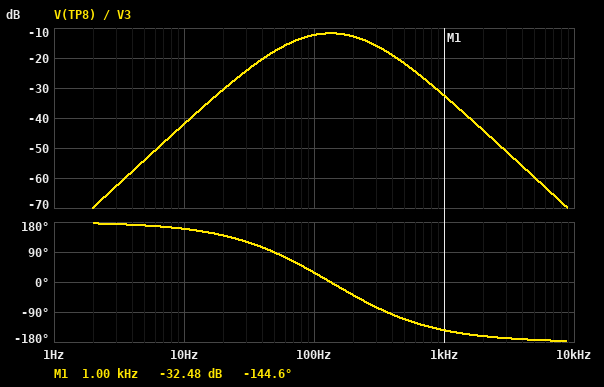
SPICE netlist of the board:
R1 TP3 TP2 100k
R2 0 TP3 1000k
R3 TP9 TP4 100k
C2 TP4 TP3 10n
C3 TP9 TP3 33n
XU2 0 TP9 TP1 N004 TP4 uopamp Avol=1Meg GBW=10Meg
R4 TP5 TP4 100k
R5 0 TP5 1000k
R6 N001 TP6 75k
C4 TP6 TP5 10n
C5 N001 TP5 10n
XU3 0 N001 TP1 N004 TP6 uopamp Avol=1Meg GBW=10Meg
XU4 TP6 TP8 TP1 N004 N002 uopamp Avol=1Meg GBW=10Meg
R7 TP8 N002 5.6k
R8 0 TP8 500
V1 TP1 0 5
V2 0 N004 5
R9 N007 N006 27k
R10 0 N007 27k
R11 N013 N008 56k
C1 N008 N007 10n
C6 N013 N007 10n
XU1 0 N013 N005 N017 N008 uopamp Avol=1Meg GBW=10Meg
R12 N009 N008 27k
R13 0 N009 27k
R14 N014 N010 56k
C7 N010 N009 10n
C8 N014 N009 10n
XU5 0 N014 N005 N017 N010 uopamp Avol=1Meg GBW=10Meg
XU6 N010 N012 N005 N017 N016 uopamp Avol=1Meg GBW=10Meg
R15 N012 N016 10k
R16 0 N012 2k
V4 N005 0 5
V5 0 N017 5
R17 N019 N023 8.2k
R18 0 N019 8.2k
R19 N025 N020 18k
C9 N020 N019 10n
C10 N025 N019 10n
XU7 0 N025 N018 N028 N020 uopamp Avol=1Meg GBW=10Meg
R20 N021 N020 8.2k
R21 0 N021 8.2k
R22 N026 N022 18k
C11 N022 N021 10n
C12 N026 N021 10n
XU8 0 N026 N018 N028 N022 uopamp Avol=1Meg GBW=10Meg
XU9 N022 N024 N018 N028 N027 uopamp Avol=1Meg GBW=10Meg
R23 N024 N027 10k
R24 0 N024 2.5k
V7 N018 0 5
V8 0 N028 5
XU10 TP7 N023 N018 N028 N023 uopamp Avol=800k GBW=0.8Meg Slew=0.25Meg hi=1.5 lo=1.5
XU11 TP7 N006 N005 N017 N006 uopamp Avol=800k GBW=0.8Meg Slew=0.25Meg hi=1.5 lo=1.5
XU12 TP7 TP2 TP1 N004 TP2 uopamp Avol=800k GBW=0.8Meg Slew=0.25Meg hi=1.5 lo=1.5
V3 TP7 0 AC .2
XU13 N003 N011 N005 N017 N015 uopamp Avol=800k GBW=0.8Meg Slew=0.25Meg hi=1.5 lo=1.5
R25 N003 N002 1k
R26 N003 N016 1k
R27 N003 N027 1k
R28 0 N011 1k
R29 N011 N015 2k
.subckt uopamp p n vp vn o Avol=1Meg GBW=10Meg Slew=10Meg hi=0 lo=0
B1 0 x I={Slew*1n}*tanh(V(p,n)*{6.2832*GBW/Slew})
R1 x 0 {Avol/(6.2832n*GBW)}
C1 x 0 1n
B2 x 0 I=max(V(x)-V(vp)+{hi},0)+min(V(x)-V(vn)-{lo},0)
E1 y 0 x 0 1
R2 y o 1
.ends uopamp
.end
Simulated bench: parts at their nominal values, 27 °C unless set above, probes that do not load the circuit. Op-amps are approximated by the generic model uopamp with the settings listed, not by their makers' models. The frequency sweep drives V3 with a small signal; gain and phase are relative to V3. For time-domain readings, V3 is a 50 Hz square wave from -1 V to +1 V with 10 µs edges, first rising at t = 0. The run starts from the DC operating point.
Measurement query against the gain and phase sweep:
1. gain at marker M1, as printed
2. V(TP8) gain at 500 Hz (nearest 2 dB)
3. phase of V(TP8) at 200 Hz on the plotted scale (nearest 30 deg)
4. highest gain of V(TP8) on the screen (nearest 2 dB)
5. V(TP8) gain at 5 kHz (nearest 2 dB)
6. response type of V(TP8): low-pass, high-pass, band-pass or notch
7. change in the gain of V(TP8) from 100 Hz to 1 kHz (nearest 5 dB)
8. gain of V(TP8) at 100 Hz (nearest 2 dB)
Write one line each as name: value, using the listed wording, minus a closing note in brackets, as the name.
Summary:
gain at marker M1, as printed: -32.48 dB
V(TP8) gain at 500 Hz: -22 dB
phase of V(TP8) at 200 Hz on the plotted scale: -30 deg
highest gain of V(TP8) on the screen: -12 dB
V(TP8) gain at 5 kHz: -60 dB
response type of V(TP8): low-pass, high-pass, band-pass or notch: band-pass
change in the gain of V(TP8) from 100 Hz to 1 kHz: -20 dB
gain of V(TP8) at 100 Hz: -12 dB
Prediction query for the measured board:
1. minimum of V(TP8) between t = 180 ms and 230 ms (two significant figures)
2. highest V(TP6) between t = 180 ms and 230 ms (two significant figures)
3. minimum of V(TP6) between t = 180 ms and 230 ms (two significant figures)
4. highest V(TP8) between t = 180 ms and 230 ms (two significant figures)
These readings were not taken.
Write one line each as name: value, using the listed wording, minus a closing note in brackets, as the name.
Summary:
minimum of V(TP8) between t = 180 ms and 230 ms: -330 mV
highest V(TP6) between t = 180 ms and 230 ms: 330 mV
minimum of V(TP6) between t = 180 ms and 230 ms: -330 mV
highest V(TP8) between t = 180 ms and 230 ms: 330 mV
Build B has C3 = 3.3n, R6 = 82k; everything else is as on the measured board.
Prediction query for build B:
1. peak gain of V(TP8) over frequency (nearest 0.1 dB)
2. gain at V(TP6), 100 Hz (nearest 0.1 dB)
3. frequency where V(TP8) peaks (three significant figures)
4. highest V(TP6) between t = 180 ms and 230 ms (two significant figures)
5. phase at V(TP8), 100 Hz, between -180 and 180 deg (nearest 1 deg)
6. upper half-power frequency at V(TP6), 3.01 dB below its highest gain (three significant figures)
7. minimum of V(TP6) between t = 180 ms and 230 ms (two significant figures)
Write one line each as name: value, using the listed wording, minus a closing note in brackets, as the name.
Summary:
peak gain of V(TP8) over frequency: -20.2 dB
gain at V(TP6), 100 Hz: -25.0 dB
frequency where V(TP8) peaks: 229 Hz
highest V(TP6) between t = 180 ms and 230 ms: 110 mV
phase at V(TP8), 100 Hz, between -180 and 180 deg: 81 deg
upper half-power frequency at V(TP6), 3.01 dB below its highest gain: 443 Hz
minimum of V(TP6) between t = 180 ms and 230 ms: -110 mV
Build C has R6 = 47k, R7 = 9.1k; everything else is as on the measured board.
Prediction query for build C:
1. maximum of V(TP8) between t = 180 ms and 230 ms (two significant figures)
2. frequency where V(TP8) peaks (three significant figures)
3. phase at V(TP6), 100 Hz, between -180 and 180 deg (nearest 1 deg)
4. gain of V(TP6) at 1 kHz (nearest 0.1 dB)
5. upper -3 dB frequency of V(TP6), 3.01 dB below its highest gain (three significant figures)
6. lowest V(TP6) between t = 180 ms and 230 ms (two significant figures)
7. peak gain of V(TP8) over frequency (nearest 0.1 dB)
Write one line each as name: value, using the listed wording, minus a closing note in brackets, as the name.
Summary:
maximum of V(TP8) between t = 180 ms and 230 ms: 210 mV
frequency where V(TP8) peaks: 137 Hz
phase at V(TP6), 100 Hz, between -180 and 180 deg: 32 deg
gain of V(TP6) at 1 kHz: -33.3 dB
upper -3 dB frequency of V(TP6), 3.01 dB below its highest gain: 295 Hz
lowest V(TP6) between t = 180 ms and 230 ms: -210 mV
peak gain of V(TP8) over frequency: -16.2 dB
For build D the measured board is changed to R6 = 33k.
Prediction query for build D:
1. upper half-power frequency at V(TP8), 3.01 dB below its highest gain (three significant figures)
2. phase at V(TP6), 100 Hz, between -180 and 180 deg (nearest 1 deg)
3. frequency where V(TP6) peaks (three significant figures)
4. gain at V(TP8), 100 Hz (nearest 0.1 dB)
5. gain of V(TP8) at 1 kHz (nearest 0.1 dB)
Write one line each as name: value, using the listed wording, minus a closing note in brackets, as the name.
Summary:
upper half-power frequency at V(TP8), 3.01 dB below its highest gain: 307 Hz
phase at V(TP6), 100 Hz, between -180 and 180 deg: 33 deg
frequency where V(TP6) peaks: 137 Hz
gain at V(TP8), 100 Hz: -20.0 dB
gain of V(TP8) at 1 kHz: -34.5 dB
